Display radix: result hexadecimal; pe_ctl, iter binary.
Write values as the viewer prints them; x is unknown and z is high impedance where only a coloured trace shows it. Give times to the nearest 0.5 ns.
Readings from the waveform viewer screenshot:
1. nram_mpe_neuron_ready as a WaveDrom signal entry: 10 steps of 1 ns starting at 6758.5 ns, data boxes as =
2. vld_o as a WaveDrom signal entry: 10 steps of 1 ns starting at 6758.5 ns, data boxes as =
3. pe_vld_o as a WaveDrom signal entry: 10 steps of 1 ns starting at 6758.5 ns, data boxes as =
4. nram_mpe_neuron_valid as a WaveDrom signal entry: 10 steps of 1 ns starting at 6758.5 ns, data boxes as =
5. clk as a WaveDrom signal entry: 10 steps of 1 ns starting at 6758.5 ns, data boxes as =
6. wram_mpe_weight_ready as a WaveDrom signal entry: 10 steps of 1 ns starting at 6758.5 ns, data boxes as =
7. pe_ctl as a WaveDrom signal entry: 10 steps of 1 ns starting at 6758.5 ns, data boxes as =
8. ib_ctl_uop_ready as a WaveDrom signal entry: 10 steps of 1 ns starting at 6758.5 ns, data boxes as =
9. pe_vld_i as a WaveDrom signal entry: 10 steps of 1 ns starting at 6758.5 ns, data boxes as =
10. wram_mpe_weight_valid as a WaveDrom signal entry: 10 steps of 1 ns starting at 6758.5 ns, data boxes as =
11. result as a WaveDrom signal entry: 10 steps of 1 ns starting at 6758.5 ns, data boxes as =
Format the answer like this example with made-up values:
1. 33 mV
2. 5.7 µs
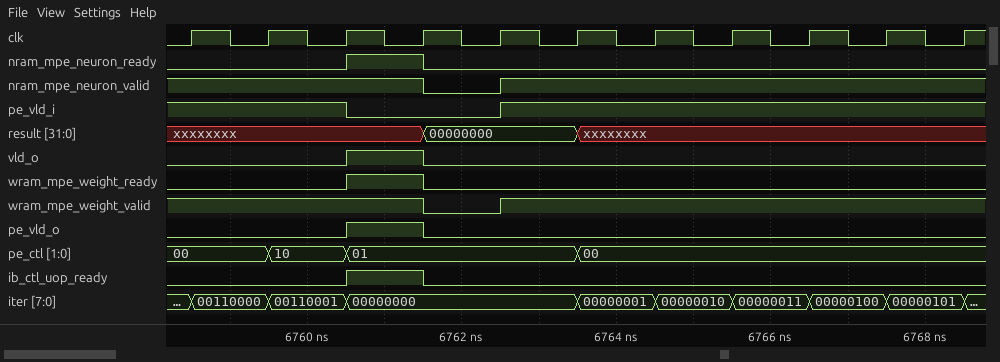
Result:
1. {name: 'nram_mpe_neuron_ready', wave: '0.10......'}
2. {name: 'vld_o', wave: '0.10......'}
3. {name: 'pe_vld_o', wave: '0.10......'}
4. {name: 'nram_mpe_neuron_valid', wave: '1..01.....'}
5. {name: 'clk', wave: 'p.........'}
6. {name: 'wram_mpe_weight_ready', wave: '0.10......'}
7. {name: 'pe_ctl', wave: '===..=....', data: '00 10 01 00'}
8. {name: 'ib_ctl_uop_ready', wave: '0.10......'}
9. {name: 'pe_vld_i', wave: '1.0.1.....'}
10. {name: 'wram_mpe_weight_valid', wave: '1..01.....'}
11. {name: 'result', wave: 'x..=.x....', data: '00000000'}
